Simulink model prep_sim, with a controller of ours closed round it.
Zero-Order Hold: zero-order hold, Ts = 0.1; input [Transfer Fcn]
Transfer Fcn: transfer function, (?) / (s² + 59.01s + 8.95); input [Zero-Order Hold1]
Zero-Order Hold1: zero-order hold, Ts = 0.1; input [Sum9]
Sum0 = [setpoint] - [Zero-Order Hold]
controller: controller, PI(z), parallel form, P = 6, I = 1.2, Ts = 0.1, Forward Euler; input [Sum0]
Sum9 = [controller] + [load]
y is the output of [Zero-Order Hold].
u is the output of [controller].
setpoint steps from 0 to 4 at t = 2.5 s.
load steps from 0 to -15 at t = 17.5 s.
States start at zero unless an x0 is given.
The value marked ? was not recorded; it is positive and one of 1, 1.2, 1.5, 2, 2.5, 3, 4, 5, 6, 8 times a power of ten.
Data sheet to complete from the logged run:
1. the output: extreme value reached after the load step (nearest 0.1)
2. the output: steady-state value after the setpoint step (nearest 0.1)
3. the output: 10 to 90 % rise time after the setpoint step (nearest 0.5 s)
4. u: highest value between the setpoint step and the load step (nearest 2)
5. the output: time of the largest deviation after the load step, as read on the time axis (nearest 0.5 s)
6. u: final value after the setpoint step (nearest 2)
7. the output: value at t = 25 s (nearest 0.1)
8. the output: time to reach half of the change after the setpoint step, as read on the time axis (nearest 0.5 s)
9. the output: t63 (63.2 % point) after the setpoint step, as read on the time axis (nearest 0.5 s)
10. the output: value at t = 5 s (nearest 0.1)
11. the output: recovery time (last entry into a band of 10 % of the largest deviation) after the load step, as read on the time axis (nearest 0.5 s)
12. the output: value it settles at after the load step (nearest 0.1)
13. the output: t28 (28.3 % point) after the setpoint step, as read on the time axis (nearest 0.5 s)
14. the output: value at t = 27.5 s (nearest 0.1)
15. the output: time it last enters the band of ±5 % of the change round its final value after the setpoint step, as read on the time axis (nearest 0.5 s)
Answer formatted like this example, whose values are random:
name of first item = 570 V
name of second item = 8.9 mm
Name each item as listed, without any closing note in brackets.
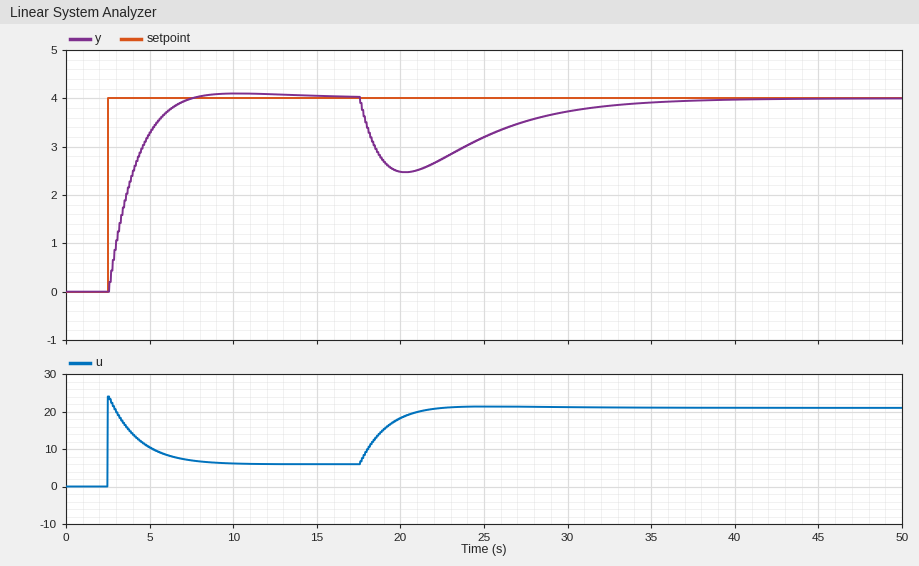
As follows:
the output: extreme value reached after the load step = 2.5
the output: steady-state value after the setpoint step = 4.0
the output: 10 to 90 % rise time after the setpoint step = 3.0 s
u: highest value between the setpoint step and the load step = 24
the output: time of the largest deviation after the load step, as read on the time axis = 20.5 s
u: final value after the setpoint step = 6
the output: value at t = 25 s = 3.2
the output: time to reach half of the change after the setpoint step, as read on the time axis = 3.5 s
the output: t63 (63.2 % point) after the setpoint step, as read on the time axis = 4.0 s
the output: value at t = 5 s = 3.3
the output: recovery time (last entry into a band of 10 % of the largest deviation) after the load step, as read on the time axis = 32.5 s
the output: value it settles at after the load step = 4.0
the output: t28 (28.3 % point) after the setpoint step, as read on the time axis = 3.0 s
the output: value at t = 27.5 s = 3.5
the output: time it last enters the band of ±5 % of the change round its final value after the setpoint step, as read on the time axis = 6.5 s
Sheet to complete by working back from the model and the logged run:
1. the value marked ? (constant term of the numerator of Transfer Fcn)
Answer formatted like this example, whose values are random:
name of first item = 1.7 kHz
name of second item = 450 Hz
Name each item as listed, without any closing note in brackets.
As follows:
the value marked ? = 6
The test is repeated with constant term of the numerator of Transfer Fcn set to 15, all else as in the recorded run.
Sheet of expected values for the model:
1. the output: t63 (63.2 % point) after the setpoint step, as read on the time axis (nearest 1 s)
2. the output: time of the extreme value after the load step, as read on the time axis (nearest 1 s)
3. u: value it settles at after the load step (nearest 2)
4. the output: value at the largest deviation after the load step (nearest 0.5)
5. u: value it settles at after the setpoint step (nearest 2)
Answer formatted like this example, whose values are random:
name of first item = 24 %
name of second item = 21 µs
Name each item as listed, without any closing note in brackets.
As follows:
the output: t63 (63.2 % point) after the setpoint step, as read on the time axis = 3 s
the output: time of the extreme value after the load step, as read on the time axis = 19 s
u: value it settles at after the load step = 18
the output: value at the largest deviation after the load step = 2.0
u: value it settles at after the setpoint step = 2
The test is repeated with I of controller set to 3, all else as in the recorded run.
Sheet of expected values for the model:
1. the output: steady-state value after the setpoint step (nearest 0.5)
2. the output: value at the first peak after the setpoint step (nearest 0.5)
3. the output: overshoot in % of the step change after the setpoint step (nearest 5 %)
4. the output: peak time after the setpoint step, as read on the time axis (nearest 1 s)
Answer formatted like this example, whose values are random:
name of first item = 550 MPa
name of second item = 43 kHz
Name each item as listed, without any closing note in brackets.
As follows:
the output: steady-state value after the setpoint step = 4.0
the output: value at the first peak after the setpoint step = 4.5
the output: overshoot in % of the step change after the setpoint step = 15 %
the output: peak time after the setpoint step, as read on the time axis = 7 s
